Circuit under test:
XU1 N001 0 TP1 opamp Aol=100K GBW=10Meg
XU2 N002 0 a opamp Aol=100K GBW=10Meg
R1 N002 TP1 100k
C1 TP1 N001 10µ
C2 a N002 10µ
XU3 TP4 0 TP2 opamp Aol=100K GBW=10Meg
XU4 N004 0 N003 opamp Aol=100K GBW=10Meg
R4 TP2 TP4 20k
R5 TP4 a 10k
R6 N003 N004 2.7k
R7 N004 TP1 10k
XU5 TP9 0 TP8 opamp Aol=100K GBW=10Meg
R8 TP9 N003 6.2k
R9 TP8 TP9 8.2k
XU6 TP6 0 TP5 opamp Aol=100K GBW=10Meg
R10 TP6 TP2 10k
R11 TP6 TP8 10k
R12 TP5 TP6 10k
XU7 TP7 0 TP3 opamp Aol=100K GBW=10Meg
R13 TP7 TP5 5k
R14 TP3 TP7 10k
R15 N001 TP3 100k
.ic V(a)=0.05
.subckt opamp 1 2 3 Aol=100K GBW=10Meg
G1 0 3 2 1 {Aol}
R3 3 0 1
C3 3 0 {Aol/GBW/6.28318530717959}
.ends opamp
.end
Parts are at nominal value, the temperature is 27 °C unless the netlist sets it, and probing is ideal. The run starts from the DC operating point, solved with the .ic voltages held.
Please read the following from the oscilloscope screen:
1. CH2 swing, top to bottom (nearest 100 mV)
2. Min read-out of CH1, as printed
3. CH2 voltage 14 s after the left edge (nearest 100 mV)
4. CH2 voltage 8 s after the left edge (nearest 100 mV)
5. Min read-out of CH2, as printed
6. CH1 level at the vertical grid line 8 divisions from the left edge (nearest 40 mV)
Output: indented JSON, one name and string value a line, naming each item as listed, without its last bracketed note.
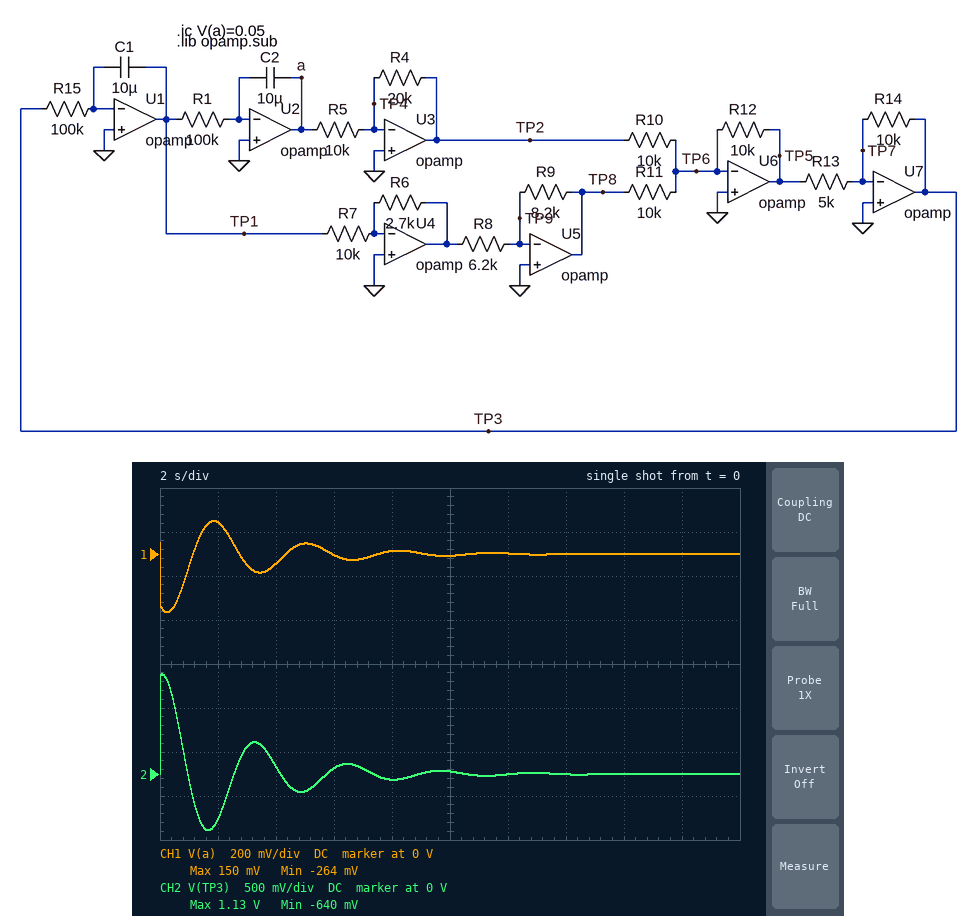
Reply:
{
  "CH2 swing, top to bottom": "1.8 V",
  "Min read-out of CH1, as printed": "-264 mV",
  "CH2 voltage 14 s after the left edge": "0 V",
  "CH2 voltage 8 s after the left edge": "-100 mV",
  "Min read-out of CH2, as printed": "-640 mV",
  "CH1 level at the vertical grid line 8 divisions from the left edge": "0 V"
}
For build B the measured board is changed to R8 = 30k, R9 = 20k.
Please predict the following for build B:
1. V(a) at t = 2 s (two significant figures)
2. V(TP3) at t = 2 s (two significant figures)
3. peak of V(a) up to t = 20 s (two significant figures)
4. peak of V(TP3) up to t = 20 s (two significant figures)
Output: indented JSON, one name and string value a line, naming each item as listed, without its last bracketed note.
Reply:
{
  "V(a) at t = 2 s": "400 mV",
  "V(TP3) at t = 2 s": "-1.5 V",
  "peak of V(a) up to t = 20 s": "430 mV",
  "peak of V(TP3) up to t = 20 s": "2.3 V"
}
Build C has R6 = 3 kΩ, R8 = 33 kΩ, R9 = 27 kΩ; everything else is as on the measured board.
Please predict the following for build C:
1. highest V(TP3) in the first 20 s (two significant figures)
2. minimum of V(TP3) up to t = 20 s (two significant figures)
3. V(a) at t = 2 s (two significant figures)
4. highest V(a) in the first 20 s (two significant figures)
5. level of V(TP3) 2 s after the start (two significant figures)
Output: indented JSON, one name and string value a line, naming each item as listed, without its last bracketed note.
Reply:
{
  "highest V(TP3) in the first 20 s": "1.7 V",
  "minimum of V(TP3) up to t = 20 s": "-1.1 V",
  "V(a) at t = 2 s": "260 mV",
  "highest V(a) in the first 20 s": "280 mV",
  "level of V(TP3) 2 s after the start": "-950 mV"
}
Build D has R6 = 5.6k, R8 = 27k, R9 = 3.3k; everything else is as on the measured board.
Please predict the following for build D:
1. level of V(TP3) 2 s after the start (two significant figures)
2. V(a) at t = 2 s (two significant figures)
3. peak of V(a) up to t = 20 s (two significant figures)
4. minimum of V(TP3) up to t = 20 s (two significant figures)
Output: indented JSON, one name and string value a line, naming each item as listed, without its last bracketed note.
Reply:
{
  "level of V(TP3) 2 s after the start": "-5.1 V",
  "V(a) at t = 2 s": "1.3 V",
  "peak of V(a) up to t = 20 s": "1.4 V",
  "minimum of V(TP3) up to t = 20 s": "-5.7 V"
}
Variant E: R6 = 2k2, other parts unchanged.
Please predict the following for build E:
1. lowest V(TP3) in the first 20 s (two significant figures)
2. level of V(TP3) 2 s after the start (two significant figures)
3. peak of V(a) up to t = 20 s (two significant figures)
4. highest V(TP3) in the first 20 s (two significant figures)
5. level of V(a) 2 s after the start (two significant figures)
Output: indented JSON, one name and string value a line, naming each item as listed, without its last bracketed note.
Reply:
{
  "lowest V(TP3) in the first 20 s": "-880 mV",
  "level of V(TP3) 2 s after the start": "-730 mV",
  "peak of V(a) up to t = 20 s": "210 mV",
  "highest V(TP3) in the first 20 s": "1.4 V",
  "level of V(a) 2 s after the start": "200 mV"
}
